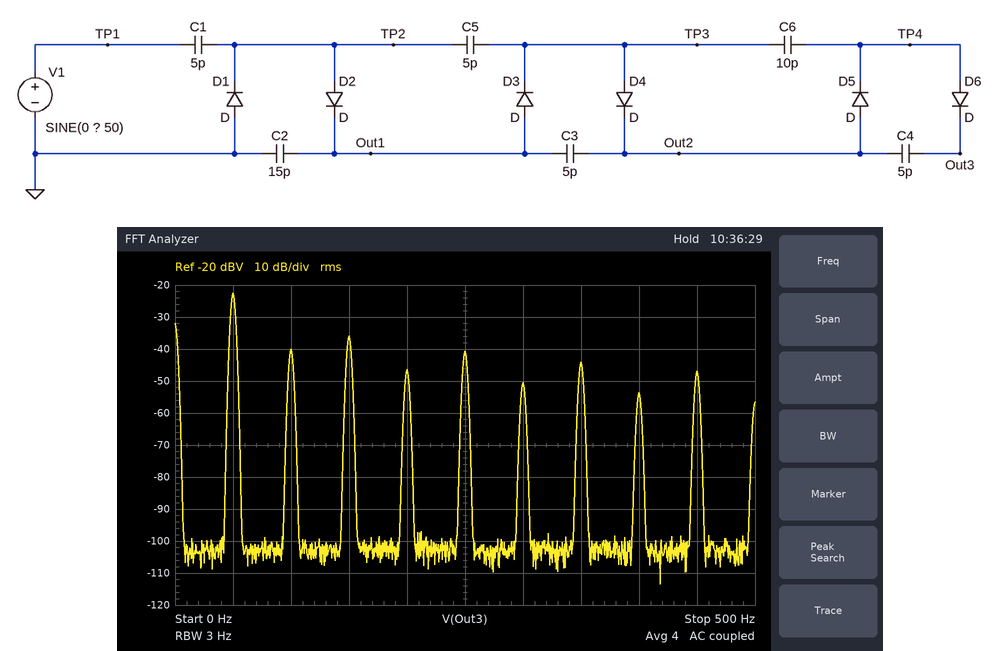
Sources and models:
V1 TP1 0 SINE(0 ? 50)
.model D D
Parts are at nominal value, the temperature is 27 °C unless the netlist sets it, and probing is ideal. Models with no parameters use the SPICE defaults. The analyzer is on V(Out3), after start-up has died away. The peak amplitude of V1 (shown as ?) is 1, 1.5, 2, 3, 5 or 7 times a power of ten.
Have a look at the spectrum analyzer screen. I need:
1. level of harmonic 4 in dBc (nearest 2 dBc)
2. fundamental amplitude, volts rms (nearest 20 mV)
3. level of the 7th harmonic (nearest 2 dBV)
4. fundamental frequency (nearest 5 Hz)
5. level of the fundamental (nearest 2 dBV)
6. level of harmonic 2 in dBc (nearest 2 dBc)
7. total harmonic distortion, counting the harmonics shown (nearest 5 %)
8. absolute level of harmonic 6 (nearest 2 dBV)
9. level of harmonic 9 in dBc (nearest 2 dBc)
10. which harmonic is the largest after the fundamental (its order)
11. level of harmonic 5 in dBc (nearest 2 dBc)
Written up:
-24 dBc
80 mV
-44 dBV
50 Hz
-22 dBV
-18 dBc
30 %
-50 dBV
-24 dBc
3
-18 dBc
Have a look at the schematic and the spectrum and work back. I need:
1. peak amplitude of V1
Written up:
10 V
